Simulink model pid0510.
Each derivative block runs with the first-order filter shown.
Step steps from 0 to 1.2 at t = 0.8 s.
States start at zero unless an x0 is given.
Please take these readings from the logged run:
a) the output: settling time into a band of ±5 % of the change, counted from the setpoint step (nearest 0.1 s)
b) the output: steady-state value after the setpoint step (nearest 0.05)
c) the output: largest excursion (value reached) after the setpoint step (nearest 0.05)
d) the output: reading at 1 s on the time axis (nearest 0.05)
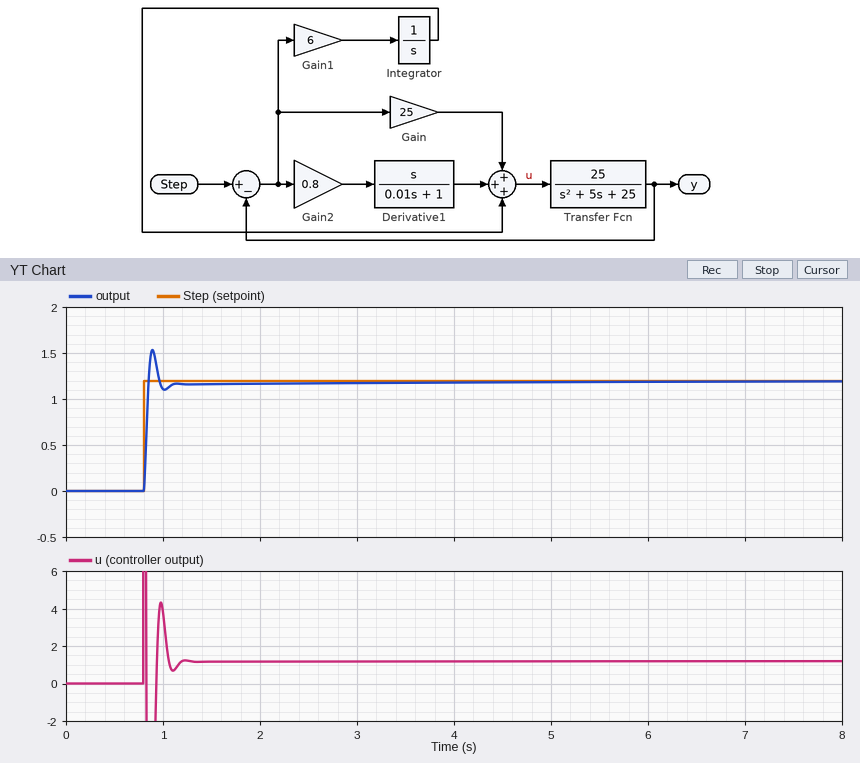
0.3 s
1.20
1.55
1.10
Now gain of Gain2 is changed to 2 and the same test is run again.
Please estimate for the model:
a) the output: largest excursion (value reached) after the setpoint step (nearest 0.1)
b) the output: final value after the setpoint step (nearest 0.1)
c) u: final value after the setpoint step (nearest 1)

1.4
1.2
1
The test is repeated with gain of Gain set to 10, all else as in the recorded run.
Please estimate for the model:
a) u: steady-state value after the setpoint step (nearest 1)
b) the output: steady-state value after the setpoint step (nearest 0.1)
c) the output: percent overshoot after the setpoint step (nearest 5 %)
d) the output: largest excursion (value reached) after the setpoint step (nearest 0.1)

1
1.2
10 %
1.3
